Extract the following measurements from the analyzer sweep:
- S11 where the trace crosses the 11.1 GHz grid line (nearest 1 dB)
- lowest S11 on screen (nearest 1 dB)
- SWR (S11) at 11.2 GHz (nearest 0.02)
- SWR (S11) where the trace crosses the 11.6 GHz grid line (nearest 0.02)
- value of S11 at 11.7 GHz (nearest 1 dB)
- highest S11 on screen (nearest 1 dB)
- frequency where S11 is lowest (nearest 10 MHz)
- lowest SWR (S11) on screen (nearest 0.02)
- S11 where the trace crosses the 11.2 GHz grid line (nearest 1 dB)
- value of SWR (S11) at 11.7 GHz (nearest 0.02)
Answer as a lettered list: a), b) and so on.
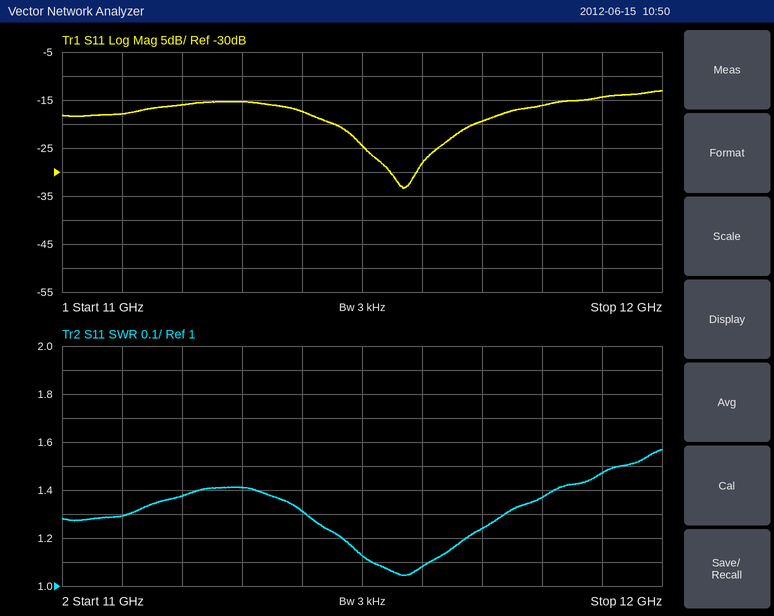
a) -18 dB
b) -33 dB
c) 1.38
d) 1.08
e) -19 dB
f) -13 dB
g) 11.57 GHz
h) 1.04
i) -16 dB
j) 1.24
